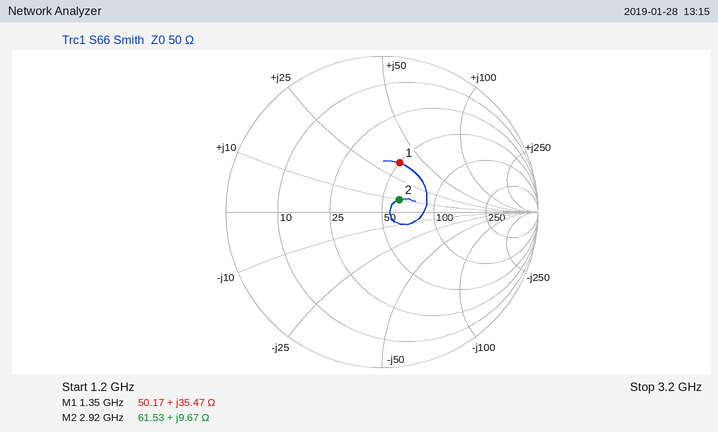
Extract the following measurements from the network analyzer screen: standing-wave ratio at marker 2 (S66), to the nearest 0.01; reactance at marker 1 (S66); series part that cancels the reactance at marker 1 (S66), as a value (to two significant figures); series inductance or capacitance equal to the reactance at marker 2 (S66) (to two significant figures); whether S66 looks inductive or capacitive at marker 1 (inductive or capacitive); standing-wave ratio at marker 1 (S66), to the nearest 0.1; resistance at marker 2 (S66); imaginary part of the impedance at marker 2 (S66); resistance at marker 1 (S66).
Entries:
1.31
+35.47 Ω
3.3 pF
530 pH
inductive
2.0
61.53 Ω
+9.67 Ω
50.17 Ω
